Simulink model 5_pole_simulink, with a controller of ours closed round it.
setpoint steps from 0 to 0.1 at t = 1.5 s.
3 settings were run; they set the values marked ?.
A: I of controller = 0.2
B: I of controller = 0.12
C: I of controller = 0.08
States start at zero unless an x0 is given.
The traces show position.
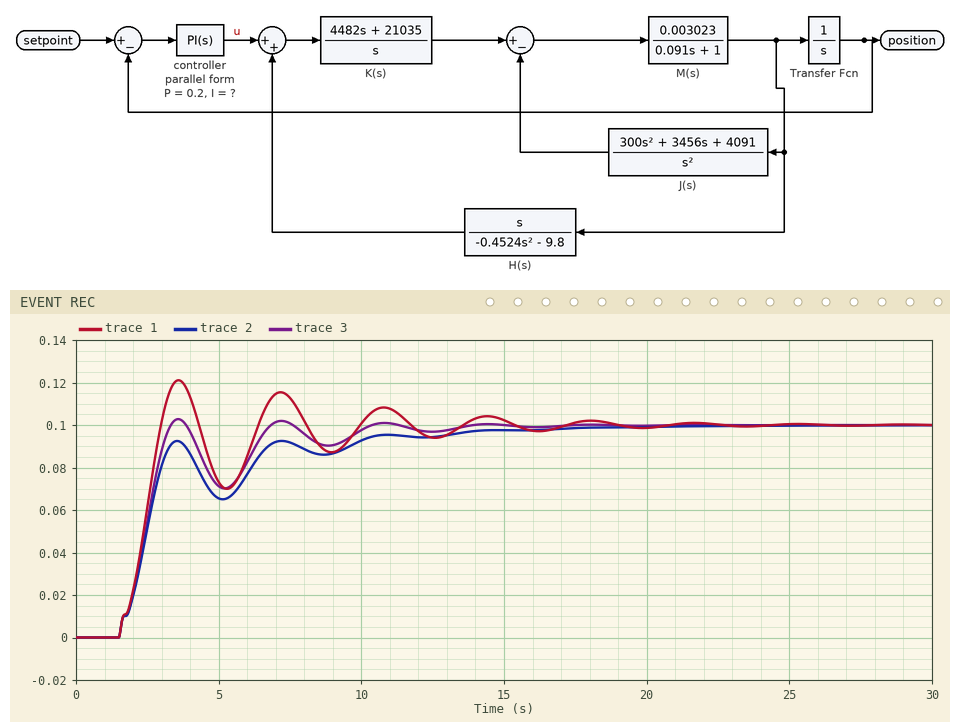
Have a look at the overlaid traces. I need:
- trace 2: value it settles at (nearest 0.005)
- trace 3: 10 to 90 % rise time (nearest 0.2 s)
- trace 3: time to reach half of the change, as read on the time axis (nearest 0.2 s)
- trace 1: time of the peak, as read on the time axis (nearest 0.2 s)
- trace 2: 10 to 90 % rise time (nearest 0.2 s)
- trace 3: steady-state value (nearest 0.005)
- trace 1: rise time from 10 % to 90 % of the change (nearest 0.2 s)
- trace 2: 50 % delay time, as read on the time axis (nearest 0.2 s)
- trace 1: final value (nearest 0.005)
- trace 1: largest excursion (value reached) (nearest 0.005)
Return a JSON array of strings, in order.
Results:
["0.100", "1.4 s", "2.4 s", "3.6 s", "1.6 s", "0.100", "1.2 s", "2.4 s", "0.100", "0.120"]
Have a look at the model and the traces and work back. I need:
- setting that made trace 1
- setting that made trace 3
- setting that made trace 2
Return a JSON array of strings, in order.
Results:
["A", "B", "C"]
